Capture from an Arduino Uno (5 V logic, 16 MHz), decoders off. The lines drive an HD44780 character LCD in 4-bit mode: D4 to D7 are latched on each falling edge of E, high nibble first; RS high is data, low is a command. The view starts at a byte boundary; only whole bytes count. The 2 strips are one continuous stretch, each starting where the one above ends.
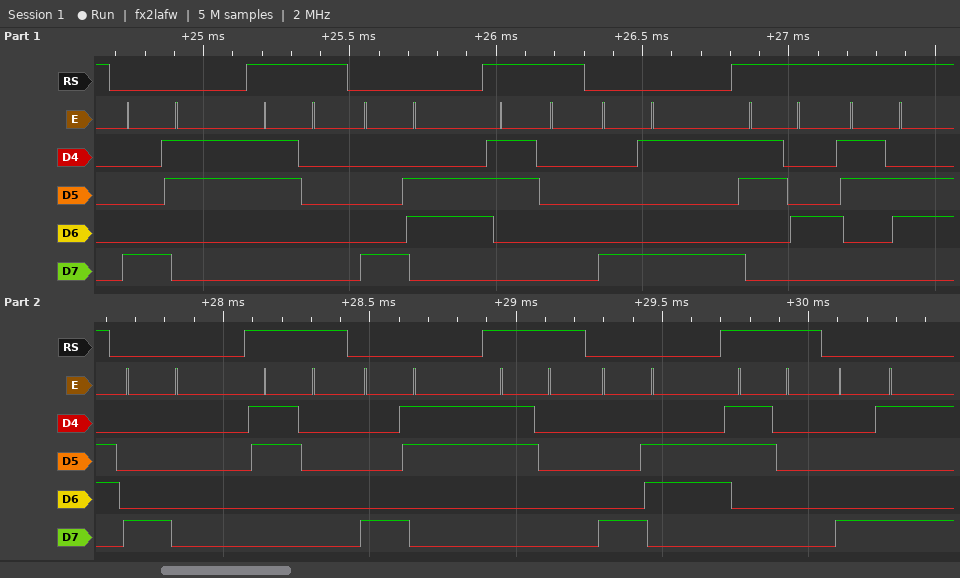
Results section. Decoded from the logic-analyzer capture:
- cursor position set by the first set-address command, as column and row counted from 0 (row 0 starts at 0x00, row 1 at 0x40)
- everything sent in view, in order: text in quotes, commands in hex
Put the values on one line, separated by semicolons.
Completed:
column 3, row 0; 0x83 "0" 0x86 "0" 0x89 "46" 0x80 "0" 0x83 "0" 0x86 "0" 0x89
